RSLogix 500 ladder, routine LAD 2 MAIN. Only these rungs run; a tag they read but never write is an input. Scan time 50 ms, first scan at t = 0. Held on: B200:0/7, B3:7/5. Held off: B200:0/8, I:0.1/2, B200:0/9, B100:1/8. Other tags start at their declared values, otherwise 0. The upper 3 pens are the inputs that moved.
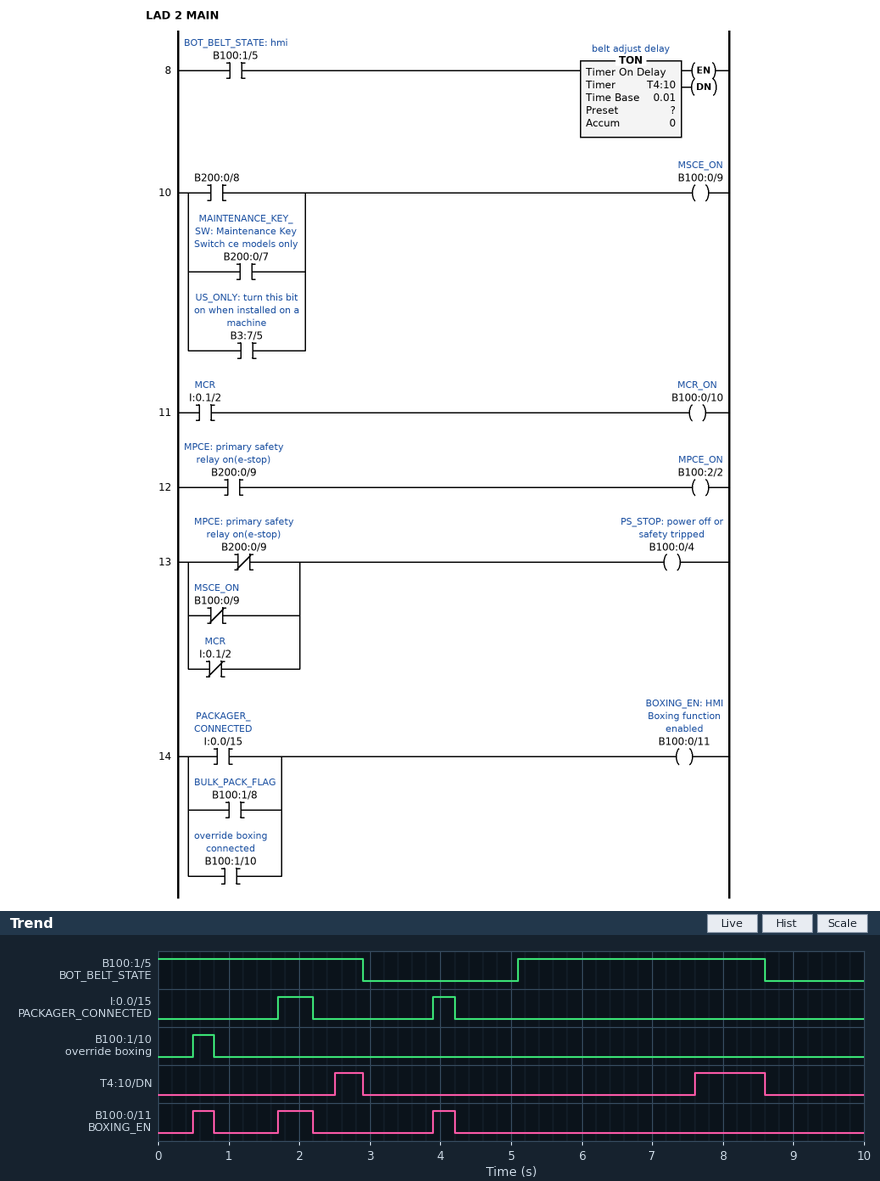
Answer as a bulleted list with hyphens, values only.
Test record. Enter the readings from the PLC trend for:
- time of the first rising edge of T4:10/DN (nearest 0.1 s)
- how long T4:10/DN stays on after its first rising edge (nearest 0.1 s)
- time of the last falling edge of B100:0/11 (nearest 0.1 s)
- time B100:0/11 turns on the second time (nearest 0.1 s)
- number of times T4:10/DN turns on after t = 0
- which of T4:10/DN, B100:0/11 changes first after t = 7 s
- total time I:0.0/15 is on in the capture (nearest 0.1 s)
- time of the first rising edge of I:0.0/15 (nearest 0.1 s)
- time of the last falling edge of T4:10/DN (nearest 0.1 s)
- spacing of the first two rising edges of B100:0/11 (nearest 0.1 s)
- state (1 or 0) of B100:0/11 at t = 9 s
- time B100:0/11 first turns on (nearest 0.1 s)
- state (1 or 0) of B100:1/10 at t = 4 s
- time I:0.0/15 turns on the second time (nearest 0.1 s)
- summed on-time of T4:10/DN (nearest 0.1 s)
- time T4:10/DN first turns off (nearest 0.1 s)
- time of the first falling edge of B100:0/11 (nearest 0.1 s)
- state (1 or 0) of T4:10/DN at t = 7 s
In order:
- 2.5 s
- 0.4 s
- 4.2 s
- 1.7 s
- 2
- T4:10/DN
- 0.8 s
- 1.7 s
- 8.6 s
- 1.2 s
- 0
- 0.5 s
- 0
- 3.9 s
- 1.4 s
- 2.9 s
- 0.8 s
- 0
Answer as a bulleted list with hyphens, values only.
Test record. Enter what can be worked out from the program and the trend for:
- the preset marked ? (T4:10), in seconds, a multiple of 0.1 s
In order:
- 2.5 s
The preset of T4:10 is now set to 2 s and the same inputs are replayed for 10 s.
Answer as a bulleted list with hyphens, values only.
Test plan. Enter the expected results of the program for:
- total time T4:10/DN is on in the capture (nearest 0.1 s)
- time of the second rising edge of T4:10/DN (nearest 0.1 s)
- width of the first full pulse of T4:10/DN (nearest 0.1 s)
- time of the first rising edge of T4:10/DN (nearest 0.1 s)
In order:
- 2.4 s
- 7.1 s
- 0.9 s
- 2.0 s
